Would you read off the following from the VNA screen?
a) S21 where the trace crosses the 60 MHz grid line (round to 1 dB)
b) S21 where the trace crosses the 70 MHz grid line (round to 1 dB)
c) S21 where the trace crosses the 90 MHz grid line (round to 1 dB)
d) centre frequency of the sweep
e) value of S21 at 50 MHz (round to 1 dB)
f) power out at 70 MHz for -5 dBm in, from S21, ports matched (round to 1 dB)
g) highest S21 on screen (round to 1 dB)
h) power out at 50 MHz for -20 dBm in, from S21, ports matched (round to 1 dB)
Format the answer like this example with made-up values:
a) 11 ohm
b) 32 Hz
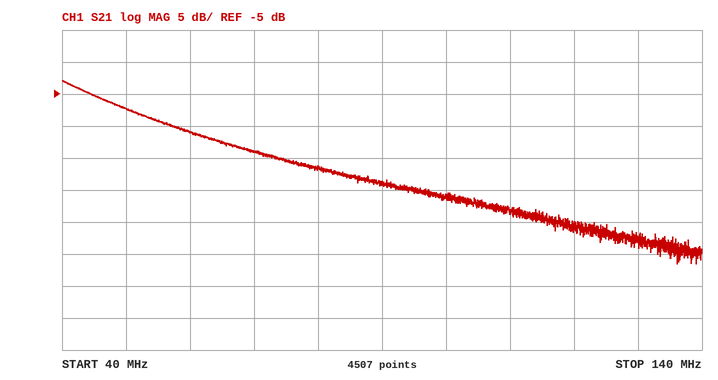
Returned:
a) -11 dB
b) -14 dB
c) -19 dB
d) 90 MHz
e) -7 dB
f) -19 dBm
g) -3 dB
h) -27 dBm
